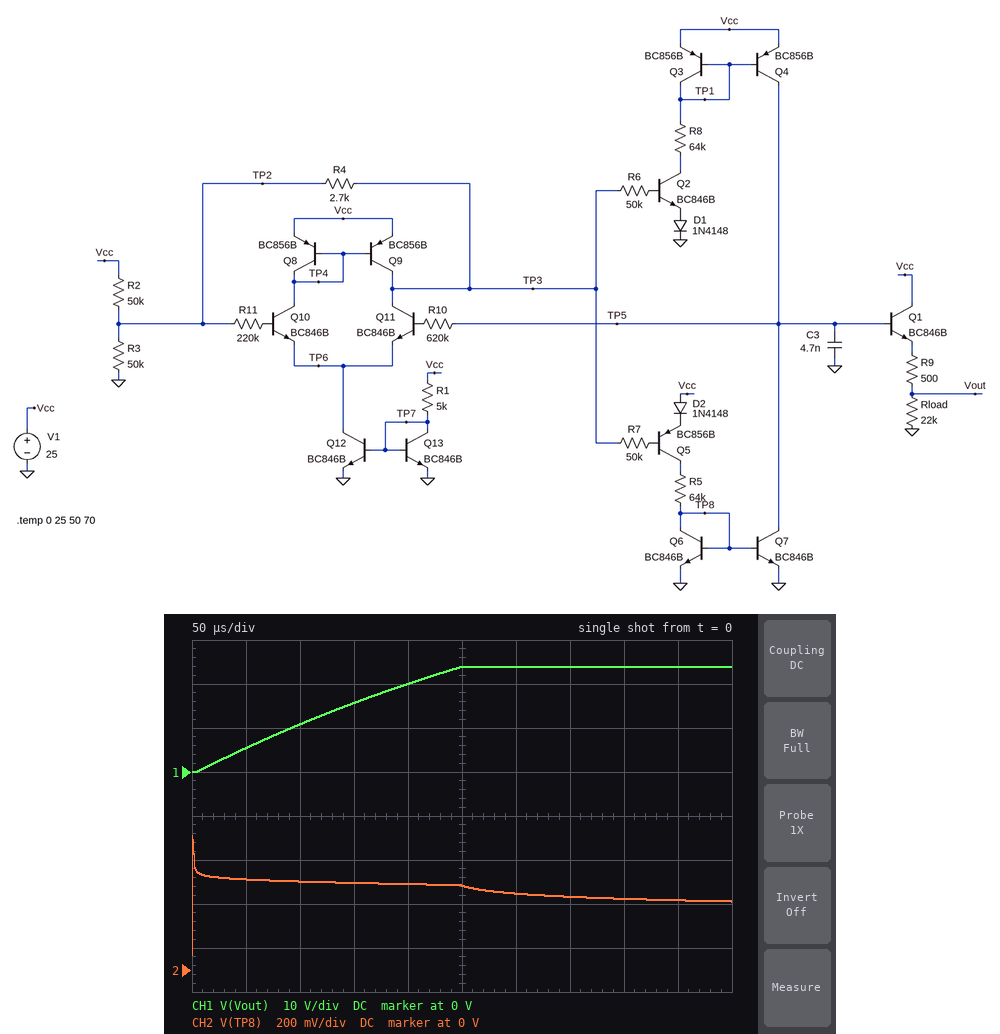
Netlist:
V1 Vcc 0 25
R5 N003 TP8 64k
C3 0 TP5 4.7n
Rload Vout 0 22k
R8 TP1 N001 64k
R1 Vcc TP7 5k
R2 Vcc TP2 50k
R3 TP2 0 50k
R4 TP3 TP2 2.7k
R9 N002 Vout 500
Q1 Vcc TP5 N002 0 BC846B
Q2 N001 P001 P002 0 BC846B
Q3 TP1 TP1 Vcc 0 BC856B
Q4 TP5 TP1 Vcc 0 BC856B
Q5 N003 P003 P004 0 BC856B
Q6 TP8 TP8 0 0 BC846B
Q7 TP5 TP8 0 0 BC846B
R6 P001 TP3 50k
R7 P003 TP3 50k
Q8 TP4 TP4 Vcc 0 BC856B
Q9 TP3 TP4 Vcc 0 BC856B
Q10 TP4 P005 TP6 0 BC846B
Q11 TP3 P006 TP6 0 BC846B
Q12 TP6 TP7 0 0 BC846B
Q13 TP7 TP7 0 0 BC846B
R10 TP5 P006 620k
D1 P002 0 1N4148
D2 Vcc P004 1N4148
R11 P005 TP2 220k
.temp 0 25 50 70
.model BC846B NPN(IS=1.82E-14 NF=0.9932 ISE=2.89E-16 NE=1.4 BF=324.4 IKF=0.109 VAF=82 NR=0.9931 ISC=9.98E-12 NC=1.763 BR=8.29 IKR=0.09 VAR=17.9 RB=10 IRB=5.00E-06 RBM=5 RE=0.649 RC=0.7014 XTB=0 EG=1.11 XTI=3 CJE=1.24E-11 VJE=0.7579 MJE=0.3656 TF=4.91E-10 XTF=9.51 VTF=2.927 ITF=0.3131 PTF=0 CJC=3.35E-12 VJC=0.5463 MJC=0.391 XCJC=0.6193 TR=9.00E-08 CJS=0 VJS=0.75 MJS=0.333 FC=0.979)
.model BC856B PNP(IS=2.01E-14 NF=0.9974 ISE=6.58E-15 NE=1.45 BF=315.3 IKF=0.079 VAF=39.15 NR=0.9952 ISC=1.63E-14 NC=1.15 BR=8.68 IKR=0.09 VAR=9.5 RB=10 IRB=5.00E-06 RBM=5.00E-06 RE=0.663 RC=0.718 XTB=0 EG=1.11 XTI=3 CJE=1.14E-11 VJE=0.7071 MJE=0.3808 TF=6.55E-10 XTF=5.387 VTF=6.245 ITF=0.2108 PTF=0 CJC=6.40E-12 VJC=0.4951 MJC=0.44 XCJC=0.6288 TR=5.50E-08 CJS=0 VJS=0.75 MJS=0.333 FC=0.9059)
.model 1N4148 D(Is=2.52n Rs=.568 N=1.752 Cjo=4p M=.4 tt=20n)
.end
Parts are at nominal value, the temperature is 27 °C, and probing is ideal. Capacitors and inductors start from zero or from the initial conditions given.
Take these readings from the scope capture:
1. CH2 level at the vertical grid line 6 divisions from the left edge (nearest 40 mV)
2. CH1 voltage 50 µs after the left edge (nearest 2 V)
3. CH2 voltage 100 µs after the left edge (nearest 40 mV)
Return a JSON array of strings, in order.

["360 mV", "6 V", "400 mV"]
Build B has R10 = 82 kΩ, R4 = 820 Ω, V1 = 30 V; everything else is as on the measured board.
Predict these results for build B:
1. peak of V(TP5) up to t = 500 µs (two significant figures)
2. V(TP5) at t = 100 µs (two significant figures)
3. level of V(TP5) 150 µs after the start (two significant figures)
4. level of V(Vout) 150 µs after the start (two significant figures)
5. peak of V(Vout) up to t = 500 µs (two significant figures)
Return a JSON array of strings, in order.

["27 V", "15 V", "21 V", "20 V", "26 V"]
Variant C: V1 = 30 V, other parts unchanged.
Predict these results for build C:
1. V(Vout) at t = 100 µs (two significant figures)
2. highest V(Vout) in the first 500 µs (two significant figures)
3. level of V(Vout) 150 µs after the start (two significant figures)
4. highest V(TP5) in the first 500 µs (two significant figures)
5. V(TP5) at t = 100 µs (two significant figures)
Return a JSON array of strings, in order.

["14 V", "29 V", "20 V", "30 V", "15 V"]
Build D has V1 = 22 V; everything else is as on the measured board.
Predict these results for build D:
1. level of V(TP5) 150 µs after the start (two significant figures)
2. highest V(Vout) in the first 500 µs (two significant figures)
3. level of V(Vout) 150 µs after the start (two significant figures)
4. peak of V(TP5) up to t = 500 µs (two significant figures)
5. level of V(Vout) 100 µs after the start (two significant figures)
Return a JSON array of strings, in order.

["14 V", "21 V", "13 V", "22 V", "9.0 V"]
